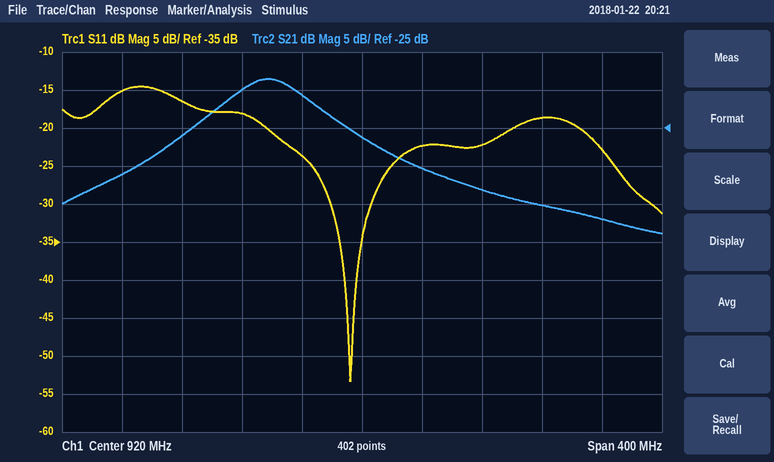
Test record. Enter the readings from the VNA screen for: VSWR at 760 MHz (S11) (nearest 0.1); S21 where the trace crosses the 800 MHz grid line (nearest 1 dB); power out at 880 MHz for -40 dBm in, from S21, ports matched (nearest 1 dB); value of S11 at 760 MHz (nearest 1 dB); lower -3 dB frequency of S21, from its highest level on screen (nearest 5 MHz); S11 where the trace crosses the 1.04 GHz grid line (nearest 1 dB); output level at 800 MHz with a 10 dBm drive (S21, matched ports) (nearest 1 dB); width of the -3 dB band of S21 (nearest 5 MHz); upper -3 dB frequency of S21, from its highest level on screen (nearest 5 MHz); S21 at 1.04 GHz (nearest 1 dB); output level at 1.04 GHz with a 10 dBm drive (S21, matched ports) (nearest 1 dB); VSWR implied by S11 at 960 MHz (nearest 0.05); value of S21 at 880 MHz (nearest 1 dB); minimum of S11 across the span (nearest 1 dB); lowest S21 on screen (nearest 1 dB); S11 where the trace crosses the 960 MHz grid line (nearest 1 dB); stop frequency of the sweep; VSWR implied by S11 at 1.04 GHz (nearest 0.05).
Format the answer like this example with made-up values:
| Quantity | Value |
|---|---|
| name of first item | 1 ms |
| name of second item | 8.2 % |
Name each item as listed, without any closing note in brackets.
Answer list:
| Quantity | Value |
|---|---|
| VSWR at 760 MHz (S11) | 1.4 |
| S21 where the trace crosses the 800 MHz grid line | -26 dB |
| power out at 880 MHz for -40 dBm in, from S21, ports matched | -61 dBm |
| value of S11 at 760 MHz | -15 dB |
| lower -3 dB frequency of S21, from its highest level on screen | 830 MHz |
| S11 where the trace crosses the 1.04 GHz grid line | -19 dB |
| output level at 800 MHz with a 10 dBm drive (S21, matched ports) | -16 dBm |
| width of the -3 dB band of S21 | 55 MHz |
| upper -3 dB frequency of S21, from its highest level on screen | 885 MHz |
| S21 at 1.04 GHz | -35 dB |
| output level at 1.04 GHz with a 10 dBm drive (S21, matched ports) | -25 dBm |
| VSWR implied by S11 at 960 MHz | 1.15 |
| value of S21 at 880 MHz | -21 dB |
| minimum of S11 across the span | -53 dB |
| lowest S21 on screen | -39 dB |
| S11 where the trace crosses the 960 MHz grid line | -22 dB |
| stop frequency of the sweep | 1.12 GHz |
| VSWR implied by S11 at 1.04 GHz | 1.25 |
